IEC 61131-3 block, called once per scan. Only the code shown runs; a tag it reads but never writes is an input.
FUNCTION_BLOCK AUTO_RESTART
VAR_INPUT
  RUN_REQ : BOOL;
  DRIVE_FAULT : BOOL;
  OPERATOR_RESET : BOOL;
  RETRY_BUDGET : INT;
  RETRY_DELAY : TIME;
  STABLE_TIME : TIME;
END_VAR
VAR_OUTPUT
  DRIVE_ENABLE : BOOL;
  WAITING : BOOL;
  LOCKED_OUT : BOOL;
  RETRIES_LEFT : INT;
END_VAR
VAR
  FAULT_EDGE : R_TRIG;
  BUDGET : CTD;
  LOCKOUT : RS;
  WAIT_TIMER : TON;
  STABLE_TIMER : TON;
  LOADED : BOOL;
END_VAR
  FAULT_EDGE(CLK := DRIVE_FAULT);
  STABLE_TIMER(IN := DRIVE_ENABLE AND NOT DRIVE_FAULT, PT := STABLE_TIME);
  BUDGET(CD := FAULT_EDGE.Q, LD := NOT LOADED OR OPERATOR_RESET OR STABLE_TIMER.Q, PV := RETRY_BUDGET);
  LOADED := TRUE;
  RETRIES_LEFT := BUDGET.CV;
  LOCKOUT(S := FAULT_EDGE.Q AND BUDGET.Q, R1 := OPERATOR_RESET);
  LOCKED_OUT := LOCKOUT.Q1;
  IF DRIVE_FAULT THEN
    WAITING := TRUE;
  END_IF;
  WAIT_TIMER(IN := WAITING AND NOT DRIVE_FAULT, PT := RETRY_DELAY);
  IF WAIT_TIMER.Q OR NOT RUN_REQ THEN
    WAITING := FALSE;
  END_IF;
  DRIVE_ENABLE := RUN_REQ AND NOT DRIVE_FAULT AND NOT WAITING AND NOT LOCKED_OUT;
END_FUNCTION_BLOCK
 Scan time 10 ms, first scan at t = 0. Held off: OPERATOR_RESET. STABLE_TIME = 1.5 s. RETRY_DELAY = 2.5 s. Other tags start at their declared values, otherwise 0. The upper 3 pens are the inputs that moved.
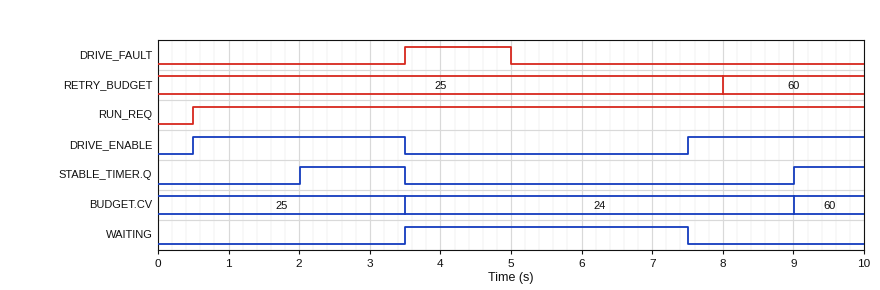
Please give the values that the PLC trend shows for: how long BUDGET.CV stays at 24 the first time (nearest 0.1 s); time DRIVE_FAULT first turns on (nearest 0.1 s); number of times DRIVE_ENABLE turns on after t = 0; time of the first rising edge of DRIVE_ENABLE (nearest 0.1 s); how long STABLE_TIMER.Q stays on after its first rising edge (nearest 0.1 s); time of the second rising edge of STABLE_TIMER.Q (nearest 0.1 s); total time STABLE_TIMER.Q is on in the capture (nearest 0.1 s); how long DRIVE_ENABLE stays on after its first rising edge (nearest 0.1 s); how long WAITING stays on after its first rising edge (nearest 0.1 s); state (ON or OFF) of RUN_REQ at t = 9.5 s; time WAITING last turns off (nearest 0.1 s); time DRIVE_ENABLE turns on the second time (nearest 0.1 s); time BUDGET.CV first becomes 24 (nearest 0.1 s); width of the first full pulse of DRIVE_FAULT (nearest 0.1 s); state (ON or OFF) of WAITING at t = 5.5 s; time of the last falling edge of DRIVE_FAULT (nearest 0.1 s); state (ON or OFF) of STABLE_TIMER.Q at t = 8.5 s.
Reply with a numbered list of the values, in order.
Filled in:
1. 5.5 s
2. 3.5 s
3. 2
4. 0.5 s
5. 1.5 s
6. 9.0 s
7. 2.5 s
8. 3.0 s
9. 4.0 s
10. ON
11. 7.5 s
12. 7.5 s
13. 3.5 s
14. 1.5 s
15. ON
16. 5.0 s
17. OFF
